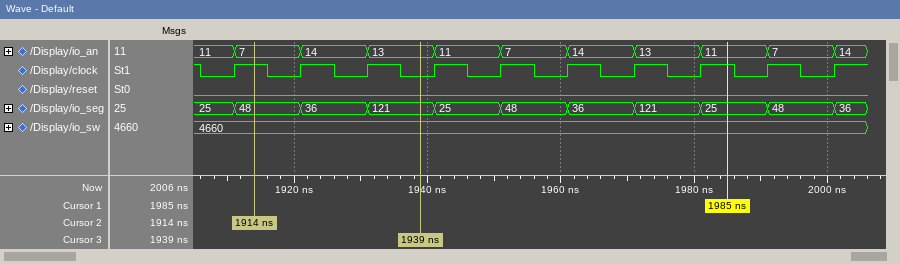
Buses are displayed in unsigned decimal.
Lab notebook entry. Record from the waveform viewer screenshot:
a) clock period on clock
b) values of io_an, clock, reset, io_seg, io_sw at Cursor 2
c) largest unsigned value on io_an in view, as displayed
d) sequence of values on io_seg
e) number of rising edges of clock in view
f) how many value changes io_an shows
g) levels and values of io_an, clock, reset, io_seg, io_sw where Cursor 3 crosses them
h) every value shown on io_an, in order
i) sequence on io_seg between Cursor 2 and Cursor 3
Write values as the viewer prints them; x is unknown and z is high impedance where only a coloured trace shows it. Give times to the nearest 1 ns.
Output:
10 ns
io_an=7, clock=1, reset=0, io_seg=48, io_sw=4660
14
25, 48, 36, 121, 25, 48, 36, 121, 25, 48, 36
10
10
io_an=13, clock=0, reset=0, io_seg=121, io_sw=4660
11, 7, 14, 13, 11, 7, 14, 13, 11, 7, 14
48, 36, 121
